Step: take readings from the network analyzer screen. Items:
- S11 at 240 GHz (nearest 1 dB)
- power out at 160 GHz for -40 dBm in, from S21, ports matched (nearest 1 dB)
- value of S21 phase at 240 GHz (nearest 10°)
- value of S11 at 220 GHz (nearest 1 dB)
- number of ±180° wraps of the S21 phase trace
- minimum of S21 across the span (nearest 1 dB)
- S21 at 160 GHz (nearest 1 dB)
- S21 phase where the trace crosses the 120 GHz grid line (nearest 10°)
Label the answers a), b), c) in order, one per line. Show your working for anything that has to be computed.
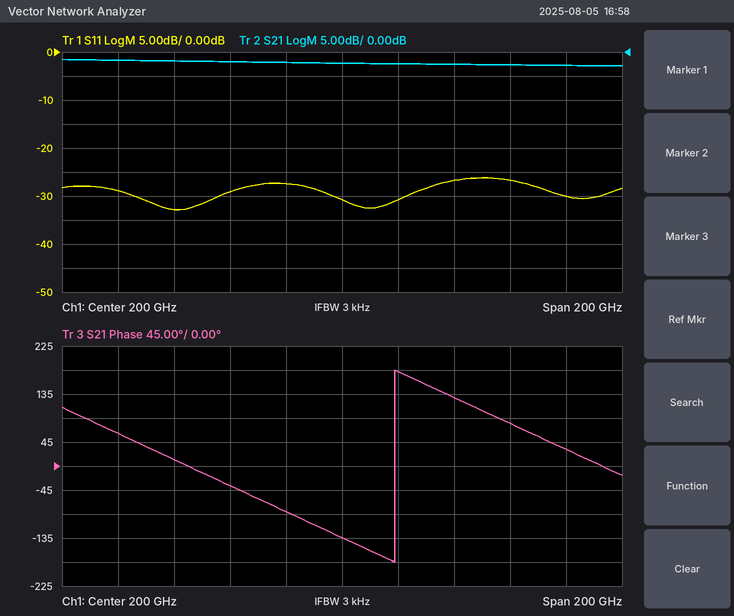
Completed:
a) -27 dB
b) -40 dBm + (-2 dB) = -42 dBm
c) 130°
d) -31 dB
e) 1
f) -3 dB
g) -2 dB
h) 60°
